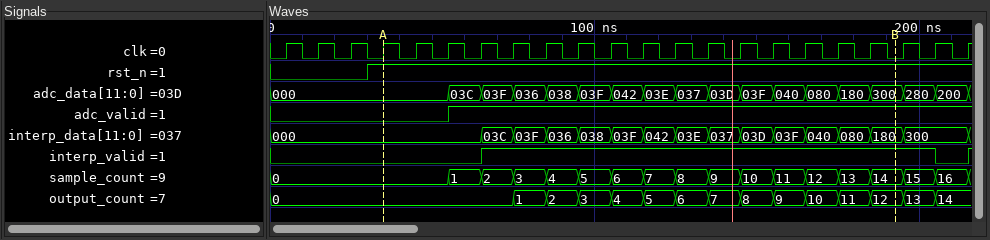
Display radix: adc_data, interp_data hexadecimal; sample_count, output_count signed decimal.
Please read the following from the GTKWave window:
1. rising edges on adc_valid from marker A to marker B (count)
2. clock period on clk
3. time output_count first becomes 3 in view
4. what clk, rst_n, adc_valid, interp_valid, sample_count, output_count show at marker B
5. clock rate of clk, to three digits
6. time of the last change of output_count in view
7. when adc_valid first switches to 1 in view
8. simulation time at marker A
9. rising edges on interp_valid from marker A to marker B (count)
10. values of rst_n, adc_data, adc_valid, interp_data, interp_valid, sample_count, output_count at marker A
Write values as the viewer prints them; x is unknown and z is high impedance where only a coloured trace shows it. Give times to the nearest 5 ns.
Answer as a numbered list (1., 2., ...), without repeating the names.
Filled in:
1. 1
2. 10 ns
3. 95 ns
4. clk=0, rst_n=1, adc_valid=1, interp_valid=1, sample_count=14, output_count=12
5. 100 MHz
6. 205 ns
7. 55 ns
8. 35 ns
9. 1
10. rst_n=1, adc_data=000, adc_valid=0, interp_data=000, interp_valid=0, sample_count=0, output_count=0
